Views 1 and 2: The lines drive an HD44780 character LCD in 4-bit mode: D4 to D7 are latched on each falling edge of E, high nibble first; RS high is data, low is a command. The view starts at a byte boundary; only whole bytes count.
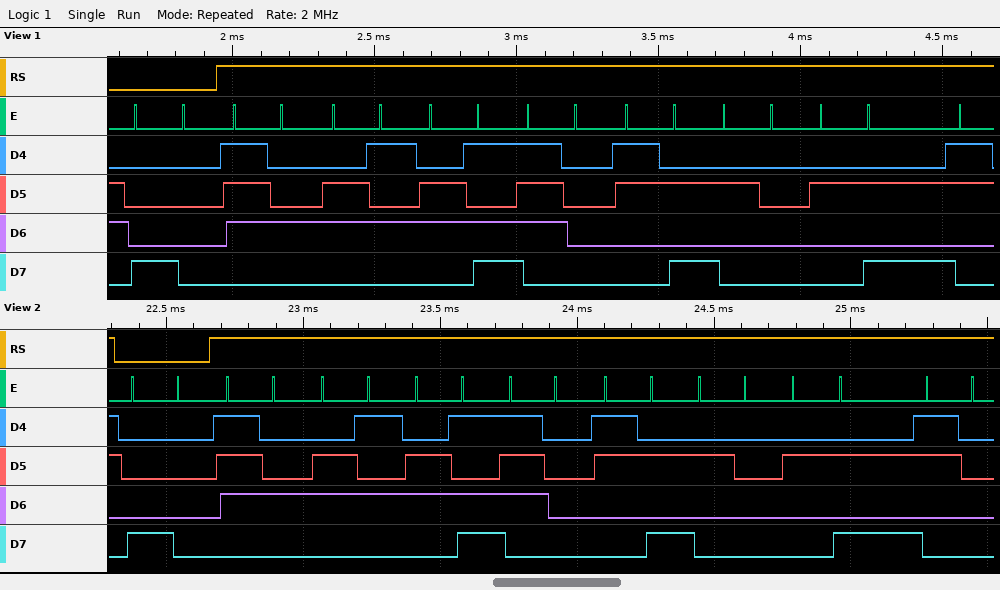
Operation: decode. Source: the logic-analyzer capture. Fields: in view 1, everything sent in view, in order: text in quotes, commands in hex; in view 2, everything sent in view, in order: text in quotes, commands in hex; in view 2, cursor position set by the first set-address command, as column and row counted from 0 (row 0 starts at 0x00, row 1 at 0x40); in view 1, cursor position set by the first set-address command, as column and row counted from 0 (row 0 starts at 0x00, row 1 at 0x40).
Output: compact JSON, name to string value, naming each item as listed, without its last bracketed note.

{"in view 1, everything sent in view, in order: text in quotes, commands in hex": "0x80 \"temp: *\"", "in view 2, everything sent in view, in order: text in quotes, commands in hex": "0x80 \"temp: *0\"", "in view 2, cursor position set by the first set-address command, as column and row counted from 0": "column 0, row 0", "in view 1, cursor position set by the first set-address command, as column and row counted from 0": "column 0, row 0"}
